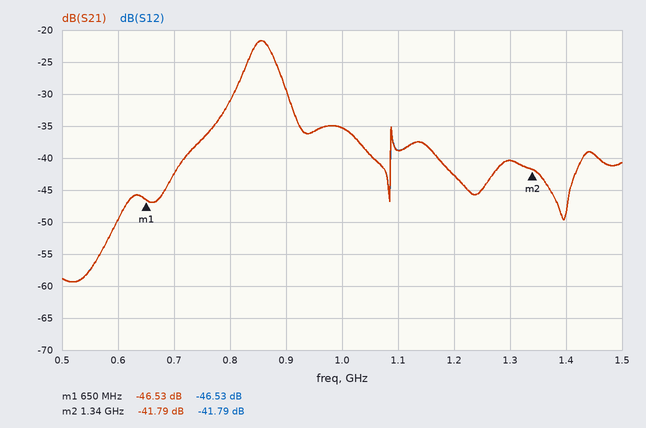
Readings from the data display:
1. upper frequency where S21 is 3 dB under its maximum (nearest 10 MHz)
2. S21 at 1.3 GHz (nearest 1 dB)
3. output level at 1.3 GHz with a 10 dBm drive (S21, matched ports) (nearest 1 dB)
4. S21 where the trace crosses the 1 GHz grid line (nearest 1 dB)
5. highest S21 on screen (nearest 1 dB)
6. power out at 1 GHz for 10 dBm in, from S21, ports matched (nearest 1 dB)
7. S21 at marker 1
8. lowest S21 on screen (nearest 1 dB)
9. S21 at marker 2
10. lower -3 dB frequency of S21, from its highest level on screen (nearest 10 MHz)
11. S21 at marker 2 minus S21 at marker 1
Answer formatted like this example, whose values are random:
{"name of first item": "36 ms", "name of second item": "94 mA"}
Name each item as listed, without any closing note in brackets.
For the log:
{"upper frequency where S21 is 3 dB under its maximum": "880 MHz", "S21 at 1.3 GHz": "-40 dB", "output level at 1.3 GHz with a 10 dBm drive (S21, matched ports)": "-30 dBm", "S21 where the trace crosses the 1 GHz grid line": "-35 dB", "highest S21 on screen": "-22 dB", "power out at 1 GHz for 10 dBm in, from S21, ports matched": "-25 dBm", "S21 at marker 1": "-46.53 dB", "lowest S21 on screen": "-59 dB", "S21 at marker 2": "-41.79 dB", "lower -3 dB frequency of S21, from its highest level on screen": "830 MHz", "S21 at marker 2 minus S21 at marker 1": "4.74 dB"}
